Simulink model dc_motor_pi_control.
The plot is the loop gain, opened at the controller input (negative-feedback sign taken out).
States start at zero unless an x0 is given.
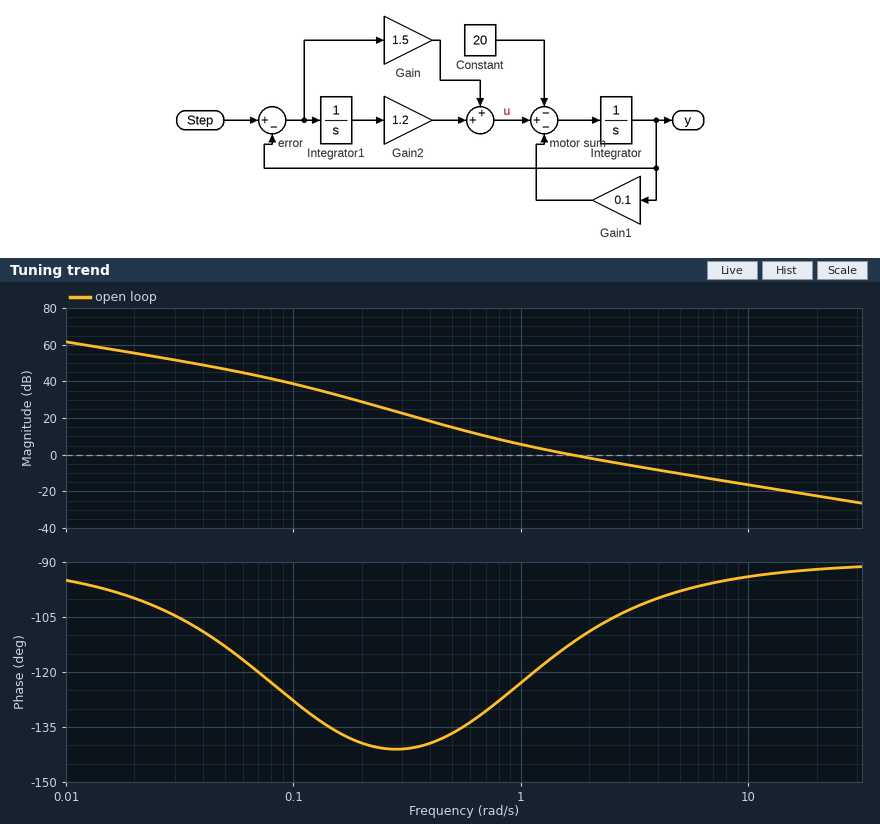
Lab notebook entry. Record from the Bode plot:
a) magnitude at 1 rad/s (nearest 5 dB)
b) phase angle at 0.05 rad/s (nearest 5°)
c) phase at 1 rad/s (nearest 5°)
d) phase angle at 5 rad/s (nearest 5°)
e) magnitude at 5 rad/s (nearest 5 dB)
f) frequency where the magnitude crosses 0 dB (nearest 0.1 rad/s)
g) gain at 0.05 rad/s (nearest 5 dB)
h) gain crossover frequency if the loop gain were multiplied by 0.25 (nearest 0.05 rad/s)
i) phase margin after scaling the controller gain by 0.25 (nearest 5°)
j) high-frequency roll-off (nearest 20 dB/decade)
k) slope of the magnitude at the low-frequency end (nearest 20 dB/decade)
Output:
5 dB
-115°
-125°
-100°
-10 dB
1.7 rad/s
45 dB
0.60 rad/s
45°
-20 dB/decade
-20 dB/decade
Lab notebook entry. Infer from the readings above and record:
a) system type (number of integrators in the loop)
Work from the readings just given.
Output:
1
